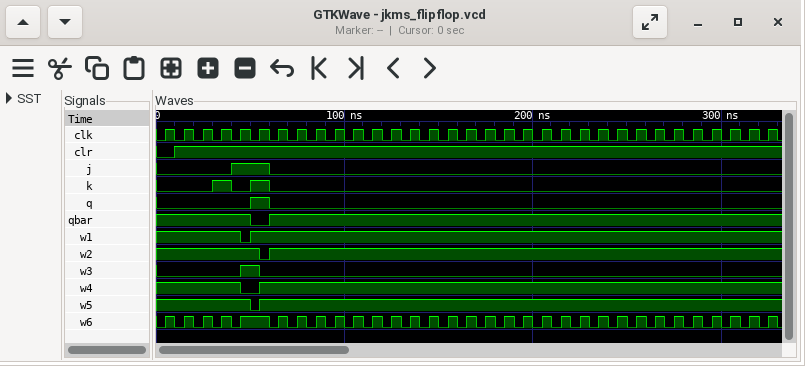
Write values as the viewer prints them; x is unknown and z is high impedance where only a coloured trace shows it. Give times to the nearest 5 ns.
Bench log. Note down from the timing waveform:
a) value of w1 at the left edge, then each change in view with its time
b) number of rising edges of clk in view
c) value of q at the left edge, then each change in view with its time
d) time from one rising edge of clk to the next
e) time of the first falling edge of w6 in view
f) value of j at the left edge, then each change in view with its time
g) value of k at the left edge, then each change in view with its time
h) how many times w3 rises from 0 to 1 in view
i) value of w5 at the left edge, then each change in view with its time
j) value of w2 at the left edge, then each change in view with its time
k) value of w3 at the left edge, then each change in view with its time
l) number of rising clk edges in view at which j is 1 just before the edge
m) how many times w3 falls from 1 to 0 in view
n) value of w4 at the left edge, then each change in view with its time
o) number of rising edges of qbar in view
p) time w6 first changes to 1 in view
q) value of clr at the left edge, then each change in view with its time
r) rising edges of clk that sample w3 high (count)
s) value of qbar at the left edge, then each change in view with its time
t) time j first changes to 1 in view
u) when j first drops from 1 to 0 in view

1, 0 at 45 ns, 1 at 50 ns
33
0, 1 at 50 ns, 0 at 60 ns
10 ns
10 ns
0, 1 at 40 ns, 0 at 60 ns
0, 1 at 30 ns, 0 at 40 ns, 1 at 50 ns, 0 at 60 ns
1
1, 0 at 50 ns, 1 at 55 ns
1, 0 at 55 ns, 1 at 60 ns
0, 1 at 45 ns, 0 at 55 ns
2
1
1, 0 at 45 ns, 1 at 55 ns
1
5 ns
0, 1 at 10 ns
1
1, 0 at 50 ns, 1 at 60 ns
40 ns
60 ns
